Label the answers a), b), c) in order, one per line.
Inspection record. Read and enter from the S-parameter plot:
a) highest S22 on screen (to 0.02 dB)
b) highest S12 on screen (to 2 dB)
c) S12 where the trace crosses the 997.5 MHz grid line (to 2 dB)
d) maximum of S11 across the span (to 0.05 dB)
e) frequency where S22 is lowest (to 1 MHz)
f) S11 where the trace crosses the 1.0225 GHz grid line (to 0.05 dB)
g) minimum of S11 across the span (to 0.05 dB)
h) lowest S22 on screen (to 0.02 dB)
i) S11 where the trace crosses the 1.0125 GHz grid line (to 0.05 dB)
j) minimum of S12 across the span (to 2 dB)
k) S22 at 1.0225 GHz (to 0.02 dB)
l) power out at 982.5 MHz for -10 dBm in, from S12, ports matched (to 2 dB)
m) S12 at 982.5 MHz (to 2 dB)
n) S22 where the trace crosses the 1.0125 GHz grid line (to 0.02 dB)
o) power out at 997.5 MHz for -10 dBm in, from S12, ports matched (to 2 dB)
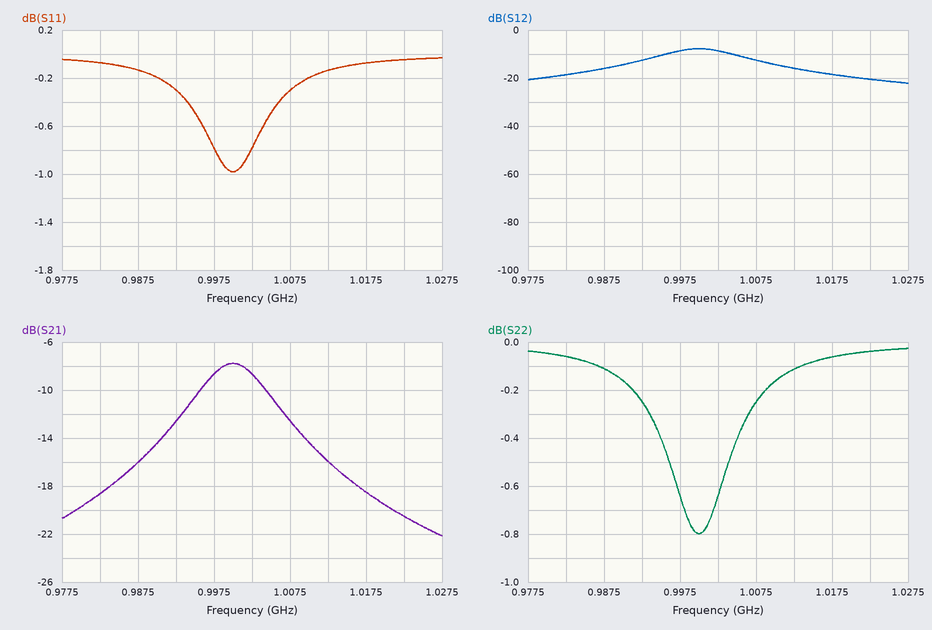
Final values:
a) -0.02 dB
b) -8 dB
c) -8 dB
d) -0.05 dB
e) 1.000 GHz
f) -0.05 dB
g) -1.00 dB
h) -0.80 dB
i) -0.15 dB
j) -22 dB
k) -0.04 dB
l) -28 dBm
m) -18 dB
n) -0.12 dB
o) -18 dBm
